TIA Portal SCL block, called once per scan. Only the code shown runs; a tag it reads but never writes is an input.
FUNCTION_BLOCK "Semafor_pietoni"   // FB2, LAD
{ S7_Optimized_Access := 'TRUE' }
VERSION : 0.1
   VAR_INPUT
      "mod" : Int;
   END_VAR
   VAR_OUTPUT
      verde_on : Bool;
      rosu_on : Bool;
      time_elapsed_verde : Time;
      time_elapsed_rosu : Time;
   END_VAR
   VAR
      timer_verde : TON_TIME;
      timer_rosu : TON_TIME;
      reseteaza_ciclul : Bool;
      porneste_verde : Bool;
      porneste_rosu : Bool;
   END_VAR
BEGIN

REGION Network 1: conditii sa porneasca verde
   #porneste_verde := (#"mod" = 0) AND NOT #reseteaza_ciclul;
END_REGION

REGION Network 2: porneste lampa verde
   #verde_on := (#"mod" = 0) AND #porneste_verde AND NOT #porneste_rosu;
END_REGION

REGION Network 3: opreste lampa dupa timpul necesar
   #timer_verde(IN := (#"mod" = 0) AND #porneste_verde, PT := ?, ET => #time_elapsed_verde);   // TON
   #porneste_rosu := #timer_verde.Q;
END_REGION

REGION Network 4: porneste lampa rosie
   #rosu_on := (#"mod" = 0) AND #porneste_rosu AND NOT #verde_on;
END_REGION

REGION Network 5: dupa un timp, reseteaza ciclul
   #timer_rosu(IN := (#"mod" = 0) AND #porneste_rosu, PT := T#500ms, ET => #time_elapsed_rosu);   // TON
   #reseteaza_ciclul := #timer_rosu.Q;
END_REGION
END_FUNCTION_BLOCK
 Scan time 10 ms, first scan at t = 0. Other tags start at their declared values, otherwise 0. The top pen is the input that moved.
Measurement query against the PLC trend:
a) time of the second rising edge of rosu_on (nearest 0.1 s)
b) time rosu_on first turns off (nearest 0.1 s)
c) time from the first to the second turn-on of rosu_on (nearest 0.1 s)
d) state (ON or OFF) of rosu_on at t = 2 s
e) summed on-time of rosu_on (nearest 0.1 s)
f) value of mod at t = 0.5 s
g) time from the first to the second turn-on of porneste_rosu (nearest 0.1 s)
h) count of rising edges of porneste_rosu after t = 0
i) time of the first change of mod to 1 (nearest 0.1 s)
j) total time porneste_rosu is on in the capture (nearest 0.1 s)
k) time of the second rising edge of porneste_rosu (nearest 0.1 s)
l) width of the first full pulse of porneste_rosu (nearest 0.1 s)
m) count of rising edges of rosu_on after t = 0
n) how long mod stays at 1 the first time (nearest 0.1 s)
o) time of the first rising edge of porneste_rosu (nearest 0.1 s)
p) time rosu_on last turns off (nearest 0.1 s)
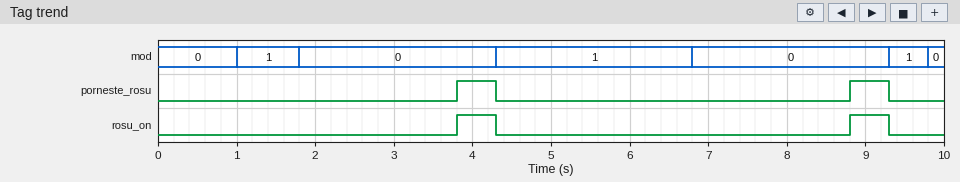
8.8 s
4.3 s
5.0 s
OFF
1.0 s
0
5.0 s
2
1.0 s
1.0 s
8.8 s
0.5 s
2
0.8 s
3.8 s
9.3 s
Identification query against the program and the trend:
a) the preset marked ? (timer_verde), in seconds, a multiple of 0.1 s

2.0 s
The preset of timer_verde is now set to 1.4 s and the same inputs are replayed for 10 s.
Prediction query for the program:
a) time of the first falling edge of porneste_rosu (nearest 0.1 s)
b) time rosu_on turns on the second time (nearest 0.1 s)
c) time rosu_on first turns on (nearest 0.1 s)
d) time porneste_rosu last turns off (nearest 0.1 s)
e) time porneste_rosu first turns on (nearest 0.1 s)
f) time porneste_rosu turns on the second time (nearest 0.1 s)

3.7 s
8.2 s
3.2 s
8.7 s
3.2 s
8.2 s
